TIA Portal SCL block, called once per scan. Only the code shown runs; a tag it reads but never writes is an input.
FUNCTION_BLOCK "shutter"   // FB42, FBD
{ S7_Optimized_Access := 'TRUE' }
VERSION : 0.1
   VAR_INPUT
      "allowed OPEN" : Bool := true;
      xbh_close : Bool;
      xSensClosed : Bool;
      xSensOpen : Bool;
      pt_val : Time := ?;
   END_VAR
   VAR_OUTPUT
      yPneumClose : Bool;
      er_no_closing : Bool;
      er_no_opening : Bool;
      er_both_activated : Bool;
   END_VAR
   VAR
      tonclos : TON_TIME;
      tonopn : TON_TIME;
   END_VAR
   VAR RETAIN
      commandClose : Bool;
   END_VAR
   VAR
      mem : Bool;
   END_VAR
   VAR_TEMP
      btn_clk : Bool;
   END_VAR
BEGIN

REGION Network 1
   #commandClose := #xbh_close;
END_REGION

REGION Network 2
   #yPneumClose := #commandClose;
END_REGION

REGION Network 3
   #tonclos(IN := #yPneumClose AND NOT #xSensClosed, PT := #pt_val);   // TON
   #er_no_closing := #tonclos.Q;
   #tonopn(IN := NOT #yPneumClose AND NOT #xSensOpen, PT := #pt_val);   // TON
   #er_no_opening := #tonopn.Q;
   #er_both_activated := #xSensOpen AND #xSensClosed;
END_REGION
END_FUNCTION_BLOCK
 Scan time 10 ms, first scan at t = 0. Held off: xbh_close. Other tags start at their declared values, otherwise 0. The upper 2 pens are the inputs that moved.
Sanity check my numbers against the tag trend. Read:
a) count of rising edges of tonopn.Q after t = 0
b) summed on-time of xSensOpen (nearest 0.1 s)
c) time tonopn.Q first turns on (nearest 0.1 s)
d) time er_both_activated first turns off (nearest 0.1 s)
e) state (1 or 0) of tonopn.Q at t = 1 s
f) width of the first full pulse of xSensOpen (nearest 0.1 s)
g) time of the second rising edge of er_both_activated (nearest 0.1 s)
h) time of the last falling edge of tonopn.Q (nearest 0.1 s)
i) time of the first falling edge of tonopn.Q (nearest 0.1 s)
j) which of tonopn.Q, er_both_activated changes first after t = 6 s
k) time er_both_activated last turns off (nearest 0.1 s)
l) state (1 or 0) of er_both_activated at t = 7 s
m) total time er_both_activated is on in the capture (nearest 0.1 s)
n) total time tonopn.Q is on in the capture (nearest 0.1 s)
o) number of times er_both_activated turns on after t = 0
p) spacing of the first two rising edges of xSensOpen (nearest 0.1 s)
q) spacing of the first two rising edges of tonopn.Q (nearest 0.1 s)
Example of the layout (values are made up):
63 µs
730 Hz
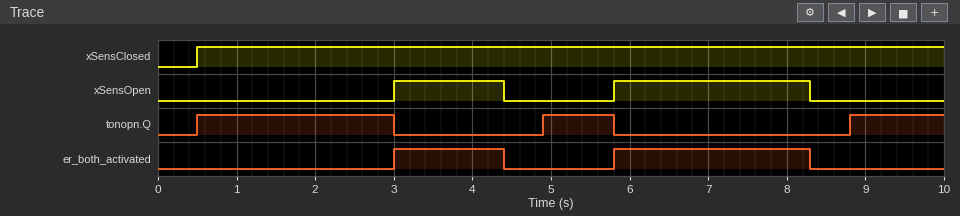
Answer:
3
3.9 s
0.5 s
4.4 s
1
1.4 s
5.8 s
5.8 s
3.0 s
er_both_activated
8.3 s
1
3.9 s
4.6 s
2
2.8 s
4.4 s
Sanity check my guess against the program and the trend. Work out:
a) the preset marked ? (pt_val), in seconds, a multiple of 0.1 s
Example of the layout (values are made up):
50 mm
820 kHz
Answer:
0.5 s
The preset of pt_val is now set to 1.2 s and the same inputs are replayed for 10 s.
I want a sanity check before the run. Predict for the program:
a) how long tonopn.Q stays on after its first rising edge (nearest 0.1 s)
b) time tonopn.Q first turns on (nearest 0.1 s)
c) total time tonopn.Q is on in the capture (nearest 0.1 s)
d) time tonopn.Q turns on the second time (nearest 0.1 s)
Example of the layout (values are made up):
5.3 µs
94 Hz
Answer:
1.8 s
1.2 s
2.5 s
5.6 s
